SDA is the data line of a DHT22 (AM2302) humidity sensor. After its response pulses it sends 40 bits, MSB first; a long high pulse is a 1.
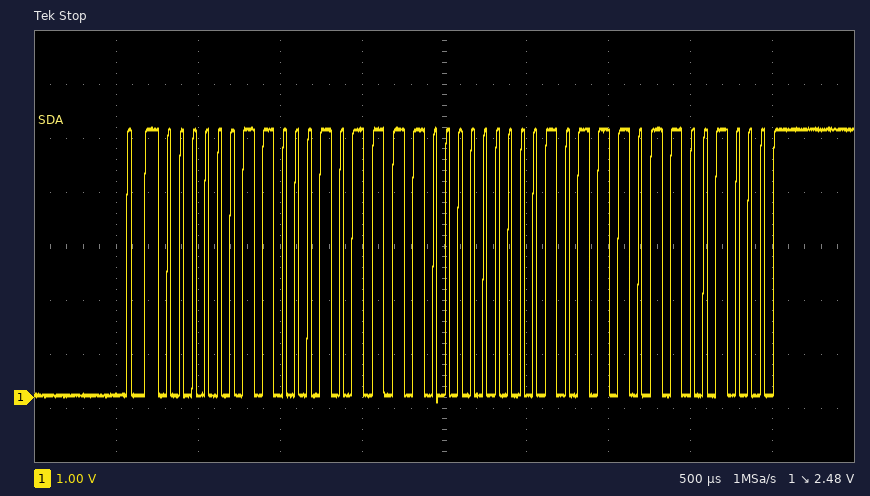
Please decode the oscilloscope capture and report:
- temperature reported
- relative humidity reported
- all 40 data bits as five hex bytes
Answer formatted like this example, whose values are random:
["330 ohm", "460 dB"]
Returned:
["-4.6 °C", "79.1 %", "03 17 80 2E C8"]
